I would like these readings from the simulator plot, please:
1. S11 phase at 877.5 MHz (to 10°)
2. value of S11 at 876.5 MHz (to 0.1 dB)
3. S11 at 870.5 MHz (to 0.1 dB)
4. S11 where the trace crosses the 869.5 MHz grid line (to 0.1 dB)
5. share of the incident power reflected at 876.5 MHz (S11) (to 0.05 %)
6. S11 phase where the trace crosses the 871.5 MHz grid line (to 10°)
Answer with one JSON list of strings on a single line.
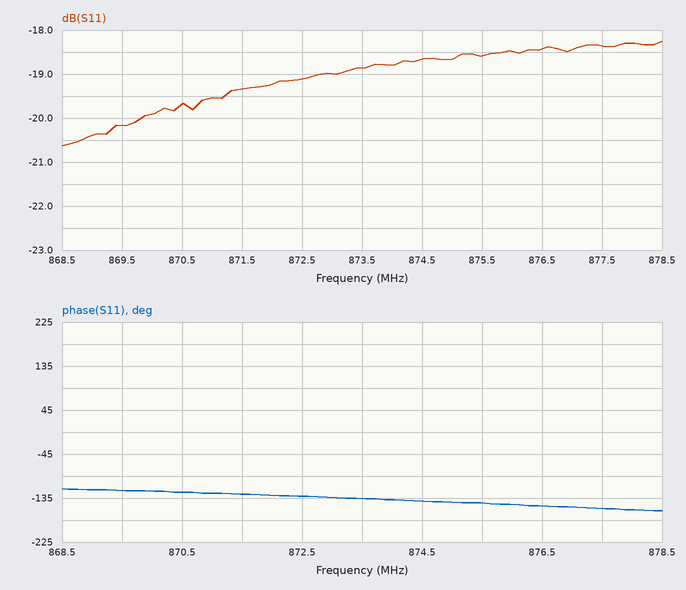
["-160°", "-18.4 dB", "-19.7 dB", "-20.2 dB", "1.45 %", "-130°"]
